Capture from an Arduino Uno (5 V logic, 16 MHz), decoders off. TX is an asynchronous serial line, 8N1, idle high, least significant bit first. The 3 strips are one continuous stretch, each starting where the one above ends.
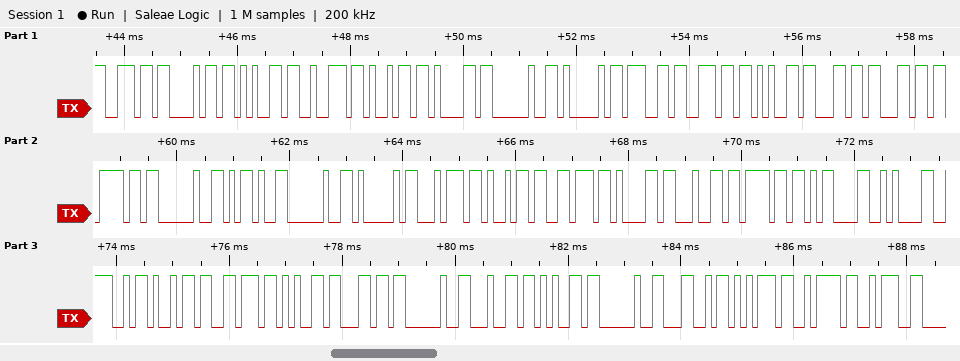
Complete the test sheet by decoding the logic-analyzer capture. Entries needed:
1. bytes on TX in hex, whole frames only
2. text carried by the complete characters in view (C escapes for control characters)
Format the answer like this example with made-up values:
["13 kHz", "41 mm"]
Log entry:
["6E 68 65 72 69 61 20 41 67 6E 65 6C 6C 6F 20 2D 20 41 74 69 76 61 64 6F 0D 0A 4E 69 76 65 6C 20 64 65 20 4C 75 7A 3A", "\"nheria Agnello - Ativado\\r\\nNivel de Luz:\""]
